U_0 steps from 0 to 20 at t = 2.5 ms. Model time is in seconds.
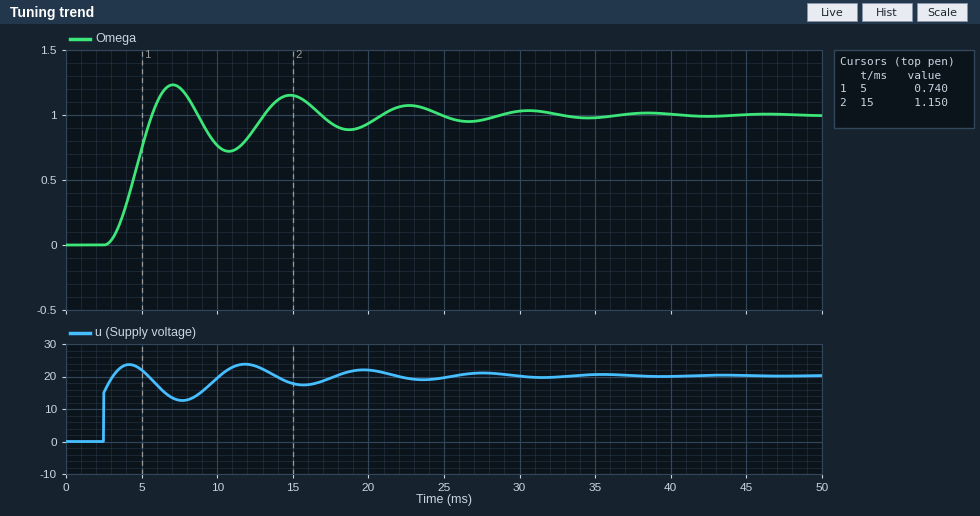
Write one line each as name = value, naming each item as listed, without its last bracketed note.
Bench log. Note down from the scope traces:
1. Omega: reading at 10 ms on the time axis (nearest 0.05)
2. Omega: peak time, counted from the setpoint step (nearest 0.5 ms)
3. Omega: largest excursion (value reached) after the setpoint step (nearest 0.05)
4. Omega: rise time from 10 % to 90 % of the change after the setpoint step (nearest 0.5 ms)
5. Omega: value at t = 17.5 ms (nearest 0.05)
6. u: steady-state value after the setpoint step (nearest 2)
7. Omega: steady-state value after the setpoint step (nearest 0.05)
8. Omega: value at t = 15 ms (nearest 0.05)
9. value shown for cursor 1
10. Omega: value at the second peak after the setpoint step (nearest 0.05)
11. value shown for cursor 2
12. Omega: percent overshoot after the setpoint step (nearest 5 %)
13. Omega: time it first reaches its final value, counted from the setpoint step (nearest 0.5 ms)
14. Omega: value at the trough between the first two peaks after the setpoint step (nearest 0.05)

Omega: reading at 10 ms on the time axis = 0.75
Omega: peak time, counted from the setpoint step = 4.5 ms
Omega: largest excursion (value reached) after the setpoint step = 1.25
Omega: rise time from 10 % to 90 % of the change after the setpoint step = 2.0 ms
Omega: value at t = 17.5 ms = 0.95
u: steady-state value after the setpoint step = 20
Omega: steady-state value after the setpoint step = 1.00
Omega: value at t = 15 ms = 1.15
value shown for cursor 1 = 0.740
Omega: value at the second peak after the setpoint step = 1.15
value shown for cursor 2 = 1.150
Omega: percent overshoot after the setpoint step = 25 %
Omega: time it first reaches its final value, counted from the setpoint step = 3.0 ms
Omega: value at the trough between the first two peaks after the setpoint step = 0.70
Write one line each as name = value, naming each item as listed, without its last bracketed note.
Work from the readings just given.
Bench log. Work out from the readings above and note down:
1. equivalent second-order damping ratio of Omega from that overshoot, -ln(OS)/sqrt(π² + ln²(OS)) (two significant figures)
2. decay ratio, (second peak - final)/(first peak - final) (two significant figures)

equivalent second-order damping ratio of Omega from that overshoot, -ln(OS)/sqrt(π² + ln²(OS)) = 0.40
decay ratio, (second peak - final)/(first peak - final) = 0.60
